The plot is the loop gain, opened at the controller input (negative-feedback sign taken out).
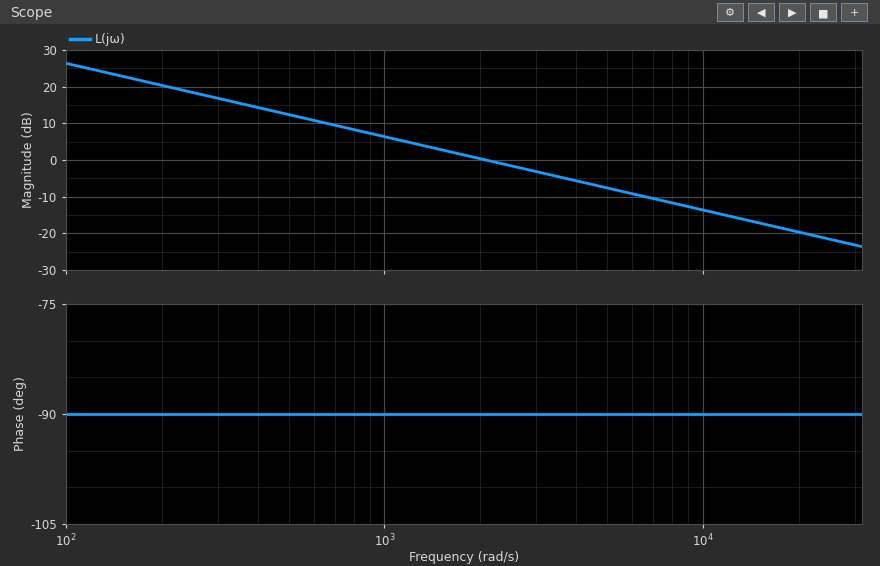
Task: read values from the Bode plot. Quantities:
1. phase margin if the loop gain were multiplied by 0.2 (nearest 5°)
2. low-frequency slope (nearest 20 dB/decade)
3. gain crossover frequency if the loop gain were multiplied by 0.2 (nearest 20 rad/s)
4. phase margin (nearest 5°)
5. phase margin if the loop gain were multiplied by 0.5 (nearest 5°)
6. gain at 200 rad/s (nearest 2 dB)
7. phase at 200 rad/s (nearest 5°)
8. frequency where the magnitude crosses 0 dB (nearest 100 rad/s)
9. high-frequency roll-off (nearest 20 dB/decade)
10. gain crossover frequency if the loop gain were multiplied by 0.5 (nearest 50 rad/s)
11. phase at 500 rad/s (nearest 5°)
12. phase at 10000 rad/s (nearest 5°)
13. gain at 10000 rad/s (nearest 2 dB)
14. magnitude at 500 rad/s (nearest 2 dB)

90°
-20 dB/decade
420 rad/s
90°
90°
20 dB
-90°
2100 rad/s
-20 dB/decade
1050 rad/s
-90°
-90°
-14 dB
12 dB
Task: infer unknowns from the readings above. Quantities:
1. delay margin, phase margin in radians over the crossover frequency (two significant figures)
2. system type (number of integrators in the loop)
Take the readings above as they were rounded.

0.00075 s
1
